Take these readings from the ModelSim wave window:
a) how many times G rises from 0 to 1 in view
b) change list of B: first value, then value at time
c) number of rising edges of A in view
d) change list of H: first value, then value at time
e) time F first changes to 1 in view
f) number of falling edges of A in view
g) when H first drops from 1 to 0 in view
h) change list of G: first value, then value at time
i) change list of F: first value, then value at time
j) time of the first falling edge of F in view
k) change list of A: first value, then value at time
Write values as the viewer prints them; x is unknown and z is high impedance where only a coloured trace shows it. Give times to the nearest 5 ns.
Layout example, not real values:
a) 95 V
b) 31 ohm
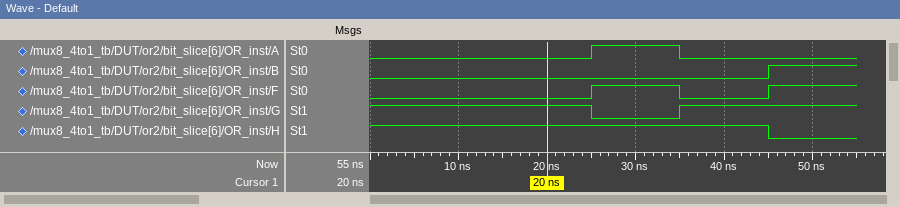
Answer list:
a) 1
b) 0, 1 at 45 ns
c) 1
d) 1, 0 at 45 ns
e) 25 ns
f) 1
g) 45 ns
h) 1, 0 at 25 ns, 1 at 35 ns
i) 0, 1 at 25 ns, 0 at 35 ns, 1 at 45 ns
j) 35 ns
k) 0, 1 at 25 ns, 0 at 35 ns
